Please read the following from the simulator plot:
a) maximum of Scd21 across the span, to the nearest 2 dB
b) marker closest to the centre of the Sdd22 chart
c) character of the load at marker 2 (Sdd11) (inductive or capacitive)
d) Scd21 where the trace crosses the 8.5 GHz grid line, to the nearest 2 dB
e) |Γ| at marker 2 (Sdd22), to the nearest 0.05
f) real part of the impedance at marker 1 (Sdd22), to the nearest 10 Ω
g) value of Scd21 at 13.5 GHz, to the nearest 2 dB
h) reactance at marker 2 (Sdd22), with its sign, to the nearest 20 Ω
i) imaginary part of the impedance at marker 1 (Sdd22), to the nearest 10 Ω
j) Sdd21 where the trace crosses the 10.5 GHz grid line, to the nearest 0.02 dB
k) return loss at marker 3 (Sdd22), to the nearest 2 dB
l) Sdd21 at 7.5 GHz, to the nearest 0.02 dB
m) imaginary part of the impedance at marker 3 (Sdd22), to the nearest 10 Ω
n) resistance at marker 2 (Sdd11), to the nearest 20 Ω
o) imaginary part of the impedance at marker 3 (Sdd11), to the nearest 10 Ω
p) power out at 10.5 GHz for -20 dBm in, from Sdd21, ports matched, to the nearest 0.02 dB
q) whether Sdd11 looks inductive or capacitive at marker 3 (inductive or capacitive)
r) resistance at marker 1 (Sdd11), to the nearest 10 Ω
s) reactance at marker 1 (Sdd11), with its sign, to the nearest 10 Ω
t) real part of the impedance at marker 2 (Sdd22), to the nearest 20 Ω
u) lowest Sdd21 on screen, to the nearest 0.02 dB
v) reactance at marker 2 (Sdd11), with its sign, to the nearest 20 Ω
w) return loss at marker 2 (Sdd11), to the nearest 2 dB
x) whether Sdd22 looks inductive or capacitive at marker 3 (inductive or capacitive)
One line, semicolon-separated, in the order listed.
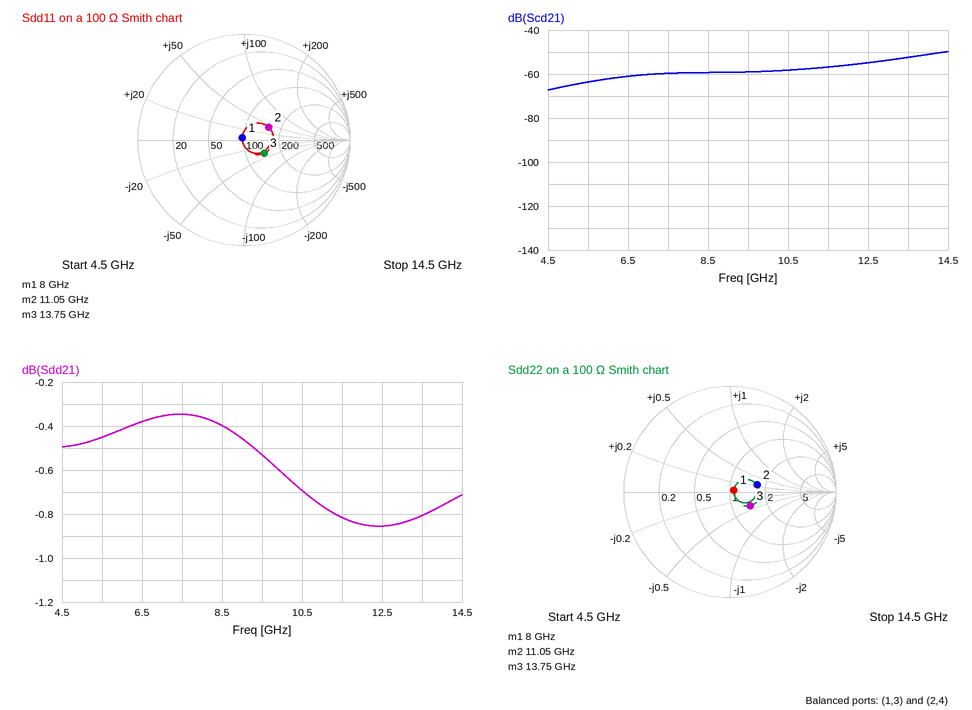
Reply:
-50 dB; marker 1; inductive; -60 dB; 0.25; 110 Ω; -52 dB; +20 Ω; 0 Ω; -0.70 dB; 12 dB; -0.34 dB; -40 Ω; 160 Ω; -40 Ω; -20.70 dBm; capacitive; 100 Ω; 0 Ω; 160 Ω; -0.86 dB; +40 Ω; 12 dB; capacitive
